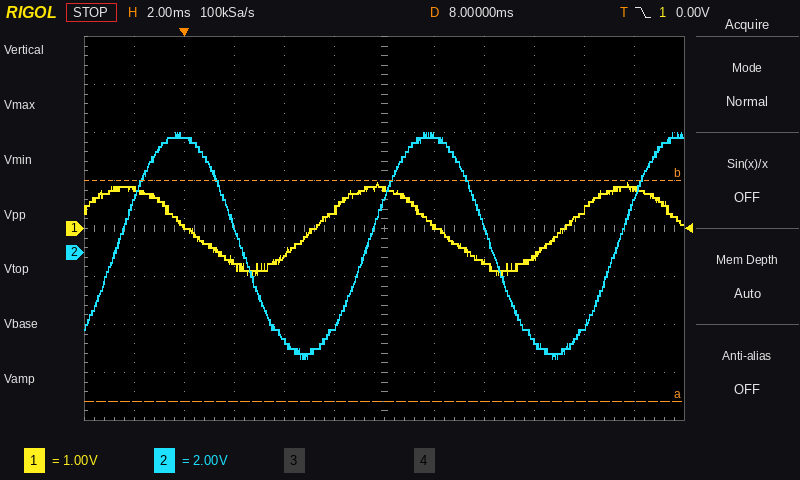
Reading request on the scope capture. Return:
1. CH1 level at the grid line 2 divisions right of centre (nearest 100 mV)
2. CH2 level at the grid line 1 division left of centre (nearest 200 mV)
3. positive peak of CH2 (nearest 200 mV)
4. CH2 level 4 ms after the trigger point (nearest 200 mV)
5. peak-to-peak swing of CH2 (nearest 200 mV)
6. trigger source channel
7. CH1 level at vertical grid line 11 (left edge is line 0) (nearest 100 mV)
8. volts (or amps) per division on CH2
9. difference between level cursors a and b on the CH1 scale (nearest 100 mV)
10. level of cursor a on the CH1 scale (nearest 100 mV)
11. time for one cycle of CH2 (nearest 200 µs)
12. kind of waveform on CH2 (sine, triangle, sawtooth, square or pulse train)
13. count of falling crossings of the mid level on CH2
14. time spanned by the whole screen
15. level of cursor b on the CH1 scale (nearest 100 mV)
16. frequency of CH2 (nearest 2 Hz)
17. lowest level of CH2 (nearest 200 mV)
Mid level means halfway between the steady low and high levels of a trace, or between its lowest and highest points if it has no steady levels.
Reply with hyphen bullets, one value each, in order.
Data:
- -700 mV
- -3.0 V
- 5.0 V
- -3.6 V
- 9.4 V
- CH1
- 800 mV
- 2 V
- 4.6 V
- -3.6 V
- 10.0 ms
- sine
- 2
- 24 ms
- 1.0 V
- 100 Hz
- -4.4 V
